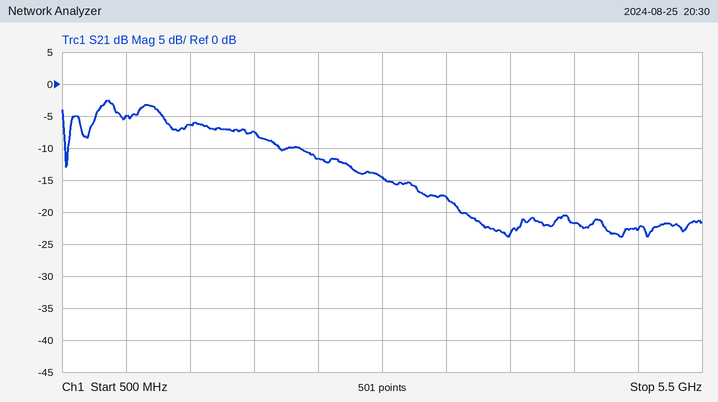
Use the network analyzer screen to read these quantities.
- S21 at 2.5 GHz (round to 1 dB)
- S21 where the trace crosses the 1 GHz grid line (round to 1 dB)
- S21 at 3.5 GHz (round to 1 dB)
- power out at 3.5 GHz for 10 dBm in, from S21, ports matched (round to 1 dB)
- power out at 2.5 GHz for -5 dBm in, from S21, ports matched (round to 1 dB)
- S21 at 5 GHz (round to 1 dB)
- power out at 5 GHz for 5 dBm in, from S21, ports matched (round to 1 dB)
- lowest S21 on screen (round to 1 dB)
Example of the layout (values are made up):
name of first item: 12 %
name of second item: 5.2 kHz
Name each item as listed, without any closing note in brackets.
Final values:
S21 at 2.5 GHz: -12 dB
S21 where the trace crosses the 1 GHz grid line: -5 dB
S21 at 3.5 GHz: -18 dB
power out at 3.5 GHz for 10 dBm in, from S21, ports matched: -8 dBm
power out at 2.5 GHz for -5 dBm in, from S21, ports matched: -17 dBm
S21 at 5 GHz: -23 dB
power out at 5 GHz for 5 dBm in, from S21, ports matched: -18 dBm
lowest S21 on screen: -24 dB
